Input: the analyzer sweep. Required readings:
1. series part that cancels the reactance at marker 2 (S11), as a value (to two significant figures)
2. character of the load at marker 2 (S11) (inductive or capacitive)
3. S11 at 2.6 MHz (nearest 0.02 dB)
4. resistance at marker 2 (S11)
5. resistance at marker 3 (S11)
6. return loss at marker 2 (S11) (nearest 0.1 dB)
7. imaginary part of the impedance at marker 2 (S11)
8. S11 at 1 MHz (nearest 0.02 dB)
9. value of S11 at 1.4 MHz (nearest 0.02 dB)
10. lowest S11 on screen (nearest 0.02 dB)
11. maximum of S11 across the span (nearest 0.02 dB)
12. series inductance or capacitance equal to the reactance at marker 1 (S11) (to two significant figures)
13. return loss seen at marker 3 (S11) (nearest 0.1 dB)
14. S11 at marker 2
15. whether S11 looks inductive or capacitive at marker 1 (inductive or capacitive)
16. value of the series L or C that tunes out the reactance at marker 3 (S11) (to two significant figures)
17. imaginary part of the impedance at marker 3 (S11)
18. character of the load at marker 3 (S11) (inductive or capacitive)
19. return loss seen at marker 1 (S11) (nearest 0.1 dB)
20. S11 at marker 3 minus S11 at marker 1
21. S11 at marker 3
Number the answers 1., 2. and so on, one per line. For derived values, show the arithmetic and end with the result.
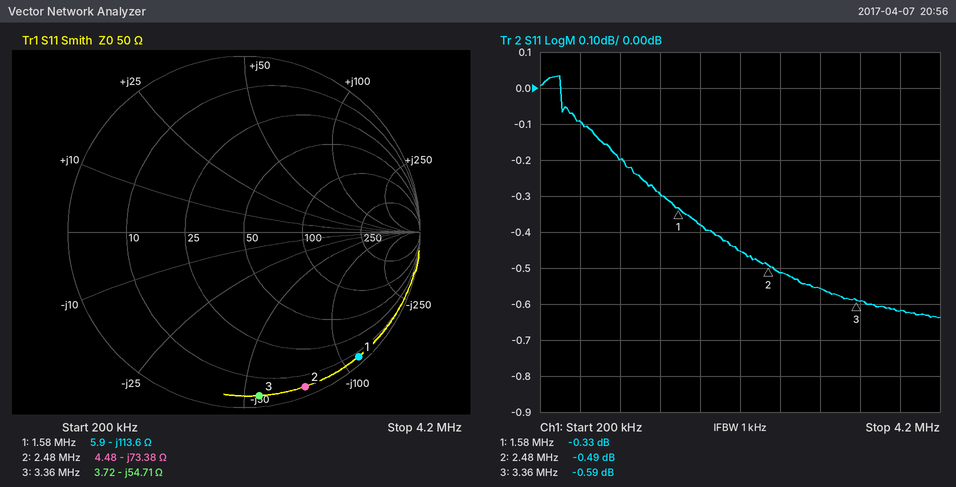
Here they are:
1. L = 73.38 Ω/(2π × 2.48 MHz) ≈ 4.7 µH
2. capacitive
3. -0.52 dB
4. 4.48 Ω
5. 3.72 Ω
6. 0.5 dB
7. -73.38 Ω
8. -0.20 dB
9. -0.30 dB
10. -0.64 dB
11. 0.04 dB
12. C = 1/(2π × 1.58 MHz × 113.6 Ω) ≈ 887 pF, so 890 pF to two significant figures
13. 0.6 dB
14. -0.49 dB
15. capacitive
16. L = 54.71 Ω/(2π × 3.36 MHz) ≈ 2.6 µH
17. -54.71 Ω
18. capacitive
19. 0.3 dB
20. -0.59 − (-0.33) = -0.26 dB
21. -0.59 dB
